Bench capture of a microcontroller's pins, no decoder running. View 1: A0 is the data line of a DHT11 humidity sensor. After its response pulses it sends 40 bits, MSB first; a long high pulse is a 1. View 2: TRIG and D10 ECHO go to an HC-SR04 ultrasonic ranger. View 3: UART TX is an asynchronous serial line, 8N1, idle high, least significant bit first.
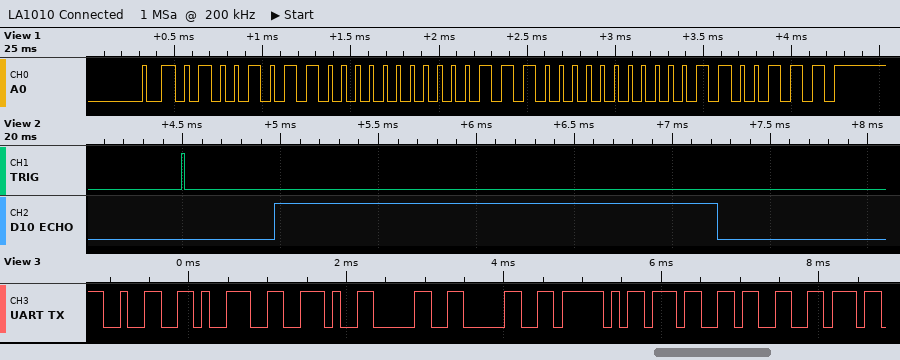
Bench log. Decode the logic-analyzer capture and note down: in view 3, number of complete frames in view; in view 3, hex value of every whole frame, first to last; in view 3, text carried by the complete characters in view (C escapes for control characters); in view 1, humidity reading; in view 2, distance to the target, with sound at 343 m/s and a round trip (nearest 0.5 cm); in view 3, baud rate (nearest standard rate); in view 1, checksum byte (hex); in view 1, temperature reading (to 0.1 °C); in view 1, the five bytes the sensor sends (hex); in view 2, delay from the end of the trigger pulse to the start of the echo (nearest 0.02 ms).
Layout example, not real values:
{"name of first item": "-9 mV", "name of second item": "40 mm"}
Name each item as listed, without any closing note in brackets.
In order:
{"in view 3, number of complete frames in view": "8", "in view 3, hex value of every whole frame, first to last": "32 39 2E 30 30 5F 37 33", "in view 3, text carried by the complete characters in view": "\"29.00_73\"", "in view 1, humidity reading": "75 %", "in view 2, distance to the target, with sound at 343 m/s and a round trip": "39 cm", "in view 3, baud rate": "9600 baud", "in view 1, checksum byte": "0x67", "in view 1, temperature reading": "28.0 °C", "in view 1, the five bytes the sensor sends": "4B 00 1C 00 67", "in view 2, delay from the end of the trigger pulse to the start of the echo": "0.46 ms"}
